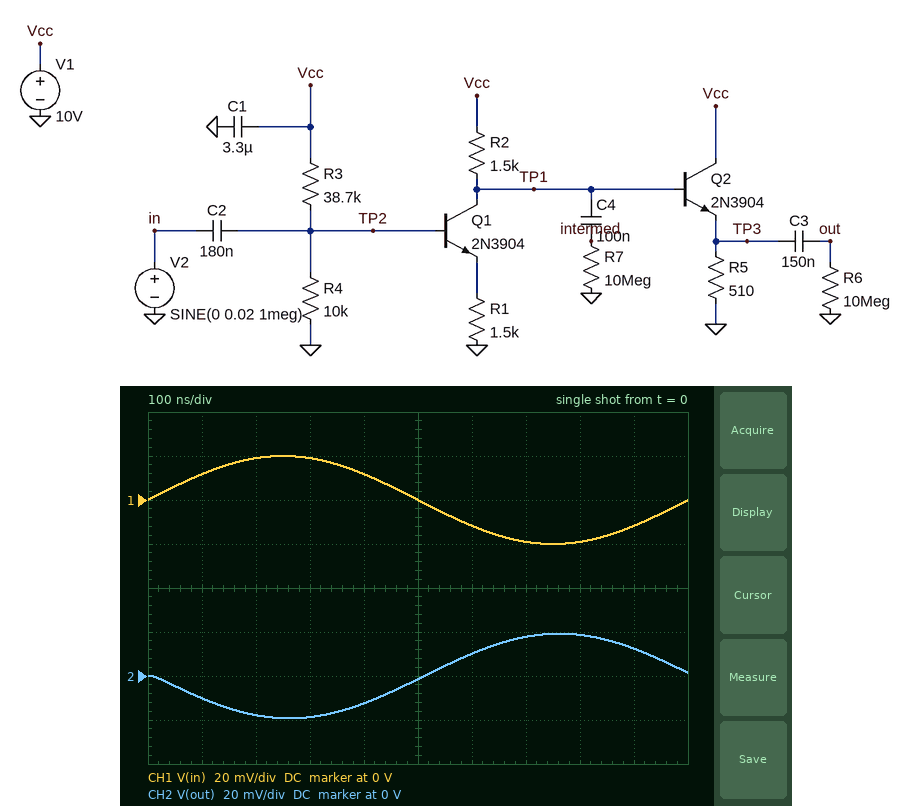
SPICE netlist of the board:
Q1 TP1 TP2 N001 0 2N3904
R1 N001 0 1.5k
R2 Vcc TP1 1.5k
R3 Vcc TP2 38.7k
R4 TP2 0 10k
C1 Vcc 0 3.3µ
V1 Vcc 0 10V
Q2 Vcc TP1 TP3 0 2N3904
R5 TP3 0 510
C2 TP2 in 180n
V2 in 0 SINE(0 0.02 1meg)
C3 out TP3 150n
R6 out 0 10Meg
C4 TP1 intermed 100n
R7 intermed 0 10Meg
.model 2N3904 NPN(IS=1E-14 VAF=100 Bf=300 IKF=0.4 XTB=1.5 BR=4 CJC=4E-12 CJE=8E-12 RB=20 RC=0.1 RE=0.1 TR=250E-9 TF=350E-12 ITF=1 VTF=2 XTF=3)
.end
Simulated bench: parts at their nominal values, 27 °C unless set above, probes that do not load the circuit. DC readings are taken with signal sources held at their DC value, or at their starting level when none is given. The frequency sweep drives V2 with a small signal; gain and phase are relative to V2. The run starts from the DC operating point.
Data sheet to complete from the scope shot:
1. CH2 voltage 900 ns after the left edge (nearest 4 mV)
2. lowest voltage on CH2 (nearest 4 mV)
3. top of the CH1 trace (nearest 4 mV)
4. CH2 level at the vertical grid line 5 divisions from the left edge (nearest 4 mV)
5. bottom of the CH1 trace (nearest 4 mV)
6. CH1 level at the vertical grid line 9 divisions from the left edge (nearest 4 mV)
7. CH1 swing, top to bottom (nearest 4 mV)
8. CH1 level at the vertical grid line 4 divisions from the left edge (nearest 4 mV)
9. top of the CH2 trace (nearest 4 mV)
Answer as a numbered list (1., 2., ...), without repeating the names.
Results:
1. 12 mV
2. -20 mV
3. 20 mV
4. 0 V
5. -20 mV
6. -12 mV
7. 40 mV
8. 12 mV
9. 20 mV
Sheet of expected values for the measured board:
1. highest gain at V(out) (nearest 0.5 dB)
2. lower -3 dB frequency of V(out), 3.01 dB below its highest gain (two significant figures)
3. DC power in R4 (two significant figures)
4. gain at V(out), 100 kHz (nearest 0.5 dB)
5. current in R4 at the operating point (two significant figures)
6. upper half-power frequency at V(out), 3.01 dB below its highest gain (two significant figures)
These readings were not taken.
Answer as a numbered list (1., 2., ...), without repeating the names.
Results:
1. -0.5 dB
2. 110 Hz
3. 410 µW
4. -0.5 dB
5. 200 µA
6. 24 MHz
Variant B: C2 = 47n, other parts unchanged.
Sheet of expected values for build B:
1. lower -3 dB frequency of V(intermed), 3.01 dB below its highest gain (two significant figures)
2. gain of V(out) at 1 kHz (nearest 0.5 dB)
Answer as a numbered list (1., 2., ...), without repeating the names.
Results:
1. 430 Hz
2. -1.0 dB
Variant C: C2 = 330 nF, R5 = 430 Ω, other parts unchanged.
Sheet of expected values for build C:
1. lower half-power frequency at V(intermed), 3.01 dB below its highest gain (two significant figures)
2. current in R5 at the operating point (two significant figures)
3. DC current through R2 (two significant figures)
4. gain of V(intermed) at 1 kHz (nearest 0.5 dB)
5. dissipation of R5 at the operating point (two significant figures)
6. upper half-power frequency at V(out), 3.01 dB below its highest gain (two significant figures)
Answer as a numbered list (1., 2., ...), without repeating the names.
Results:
1. 62 Hz
2. 18 mA
3. 980 µA
4. -0.5 dB
5. 140 mW
6. 23 MHz
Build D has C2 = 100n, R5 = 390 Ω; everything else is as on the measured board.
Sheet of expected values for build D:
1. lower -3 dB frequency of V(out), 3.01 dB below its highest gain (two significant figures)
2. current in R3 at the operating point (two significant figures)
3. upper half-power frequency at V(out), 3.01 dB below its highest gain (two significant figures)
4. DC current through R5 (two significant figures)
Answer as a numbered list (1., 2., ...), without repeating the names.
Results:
1. 200 Hz
2. 210 µA
3. 23 MHz
4. 20 mA
